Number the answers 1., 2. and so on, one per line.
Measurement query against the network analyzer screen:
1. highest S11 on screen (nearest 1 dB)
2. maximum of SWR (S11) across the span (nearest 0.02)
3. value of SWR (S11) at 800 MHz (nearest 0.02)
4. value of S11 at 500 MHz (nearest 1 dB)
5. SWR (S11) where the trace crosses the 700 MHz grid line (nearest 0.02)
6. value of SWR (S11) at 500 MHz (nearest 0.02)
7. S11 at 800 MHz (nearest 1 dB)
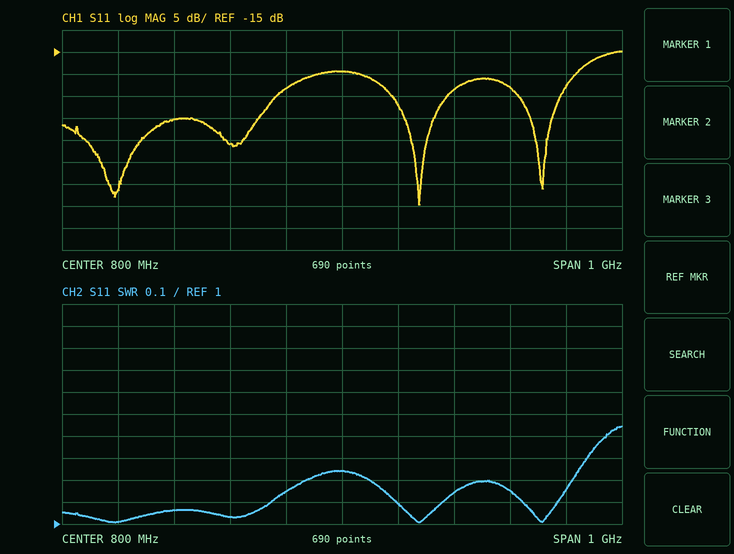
1. -15 dB
2. 1.44
3. 1.24
4. -30 dB
5. 1.14
6. 1.06
7. -19 dB
